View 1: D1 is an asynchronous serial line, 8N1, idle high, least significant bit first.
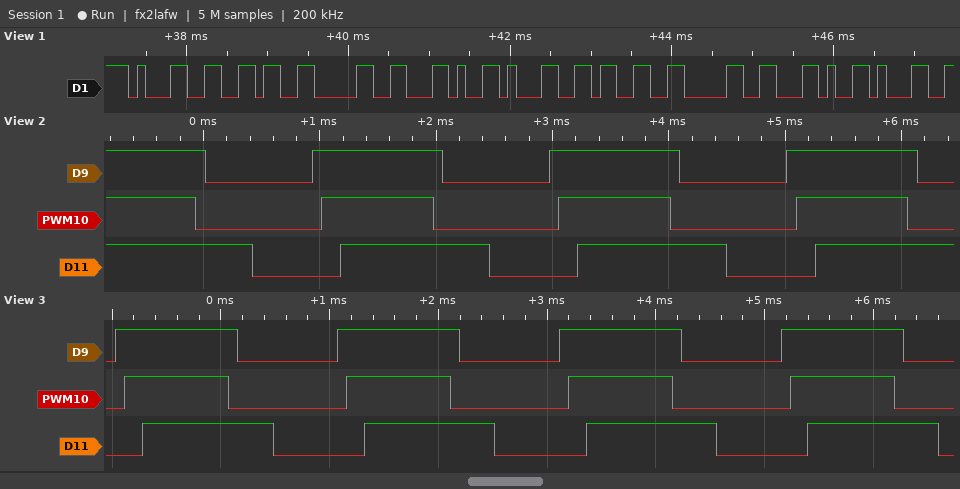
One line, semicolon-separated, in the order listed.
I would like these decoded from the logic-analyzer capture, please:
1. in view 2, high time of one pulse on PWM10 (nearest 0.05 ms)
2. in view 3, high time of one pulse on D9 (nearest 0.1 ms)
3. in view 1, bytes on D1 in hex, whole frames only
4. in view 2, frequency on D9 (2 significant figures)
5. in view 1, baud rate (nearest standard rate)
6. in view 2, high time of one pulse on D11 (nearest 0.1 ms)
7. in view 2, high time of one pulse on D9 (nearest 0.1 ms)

0.95 ms; 1.1 ms; 31 36 30 2C 31 33 30 2C 31; 490 Hz; 9600 baud; 1.3 ms; 1.1 ms
